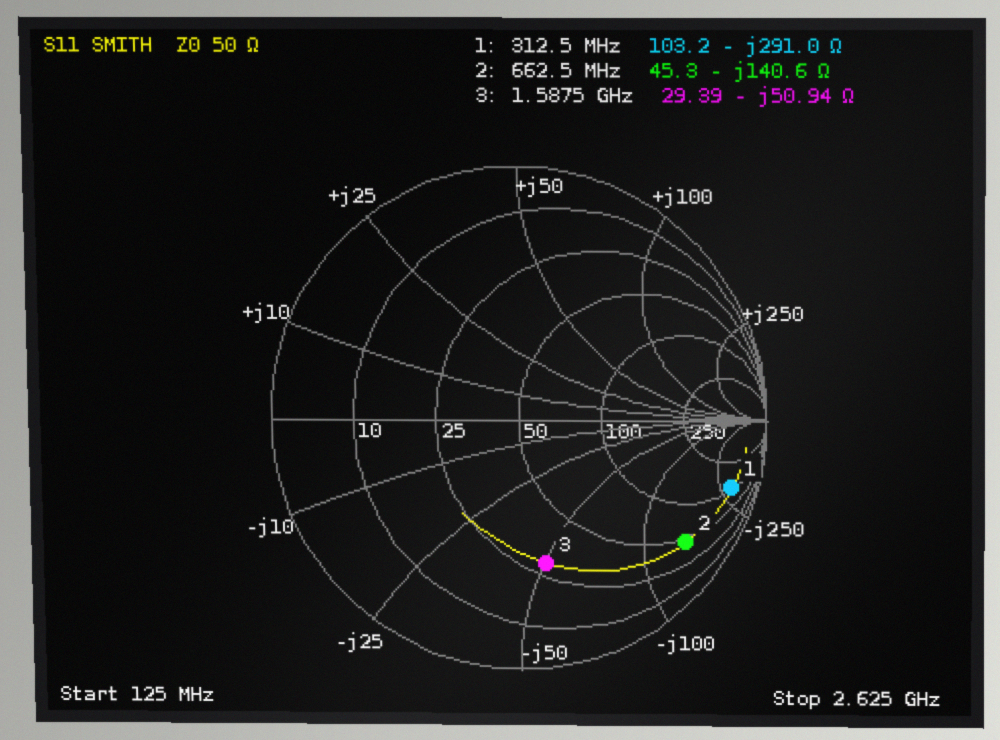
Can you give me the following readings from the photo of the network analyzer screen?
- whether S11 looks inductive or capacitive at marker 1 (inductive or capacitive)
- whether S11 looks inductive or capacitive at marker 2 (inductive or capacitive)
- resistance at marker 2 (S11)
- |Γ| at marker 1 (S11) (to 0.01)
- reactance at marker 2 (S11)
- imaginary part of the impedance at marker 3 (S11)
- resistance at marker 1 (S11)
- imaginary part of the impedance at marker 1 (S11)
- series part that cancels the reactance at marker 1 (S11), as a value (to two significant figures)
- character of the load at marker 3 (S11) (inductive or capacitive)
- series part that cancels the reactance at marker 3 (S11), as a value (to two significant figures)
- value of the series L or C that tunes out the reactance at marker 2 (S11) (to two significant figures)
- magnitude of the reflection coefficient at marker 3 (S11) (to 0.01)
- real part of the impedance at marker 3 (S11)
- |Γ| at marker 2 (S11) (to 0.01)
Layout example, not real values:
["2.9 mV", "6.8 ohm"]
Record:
["capacitive", "capacitive", "45.3 Ω", "0.90", "-140.6 Ω", "-50.94 Ω", "103.2 Ω", "-291.0 Ω", "150 nH", "capacitive", "5.1 nH", "34 nH", "0.58", "29.39 Ω", "0.83"]
